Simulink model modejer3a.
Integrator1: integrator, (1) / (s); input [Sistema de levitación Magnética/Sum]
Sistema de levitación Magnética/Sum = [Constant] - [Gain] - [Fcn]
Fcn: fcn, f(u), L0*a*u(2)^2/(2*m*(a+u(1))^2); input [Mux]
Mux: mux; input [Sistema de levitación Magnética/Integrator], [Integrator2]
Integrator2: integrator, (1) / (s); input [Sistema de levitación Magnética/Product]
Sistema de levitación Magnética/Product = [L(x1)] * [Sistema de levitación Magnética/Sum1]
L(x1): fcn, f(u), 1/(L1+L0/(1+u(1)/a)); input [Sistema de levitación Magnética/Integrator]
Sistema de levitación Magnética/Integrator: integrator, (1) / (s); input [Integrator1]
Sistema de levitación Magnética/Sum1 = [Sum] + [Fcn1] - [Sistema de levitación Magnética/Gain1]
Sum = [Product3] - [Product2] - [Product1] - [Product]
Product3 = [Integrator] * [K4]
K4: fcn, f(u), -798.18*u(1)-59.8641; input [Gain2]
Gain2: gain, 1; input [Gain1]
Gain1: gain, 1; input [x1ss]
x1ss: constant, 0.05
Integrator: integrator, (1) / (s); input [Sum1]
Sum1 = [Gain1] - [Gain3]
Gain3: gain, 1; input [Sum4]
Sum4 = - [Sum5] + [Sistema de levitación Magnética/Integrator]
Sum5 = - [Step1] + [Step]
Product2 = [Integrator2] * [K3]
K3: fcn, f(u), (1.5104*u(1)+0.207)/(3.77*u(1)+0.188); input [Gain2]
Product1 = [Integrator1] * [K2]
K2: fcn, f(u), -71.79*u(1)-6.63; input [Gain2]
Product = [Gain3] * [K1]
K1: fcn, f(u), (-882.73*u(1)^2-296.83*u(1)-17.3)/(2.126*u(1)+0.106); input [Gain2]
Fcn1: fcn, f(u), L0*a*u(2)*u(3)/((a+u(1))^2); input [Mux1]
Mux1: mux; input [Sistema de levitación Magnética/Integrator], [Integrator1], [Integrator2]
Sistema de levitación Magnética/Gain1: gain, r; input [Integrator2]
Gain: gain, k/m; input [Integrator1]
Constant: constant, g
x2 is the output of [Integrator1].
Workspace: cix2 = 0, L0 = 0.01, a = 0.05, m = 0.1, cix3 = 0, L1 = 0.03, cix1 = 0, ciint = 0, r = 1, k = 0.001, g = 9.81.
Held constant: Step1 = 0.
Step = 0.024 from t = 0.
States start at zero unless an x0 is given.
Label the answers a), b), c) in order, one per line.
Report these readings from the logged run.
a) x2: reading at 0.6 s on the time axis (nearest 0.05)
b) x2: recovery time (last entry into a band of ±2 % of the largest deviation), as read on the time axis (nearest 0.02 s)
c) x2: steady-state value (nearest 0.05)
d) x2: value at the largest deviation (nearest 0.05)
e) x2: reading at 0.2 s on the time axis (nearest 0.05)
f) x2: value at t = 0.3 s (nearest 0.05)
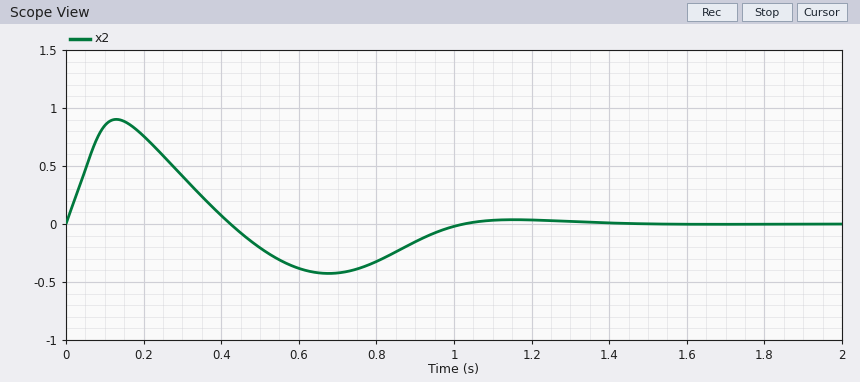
a) -0.40
b) 1.32 s
c) 0.00
d) 0.90
e) 0.75
f) 0.40
